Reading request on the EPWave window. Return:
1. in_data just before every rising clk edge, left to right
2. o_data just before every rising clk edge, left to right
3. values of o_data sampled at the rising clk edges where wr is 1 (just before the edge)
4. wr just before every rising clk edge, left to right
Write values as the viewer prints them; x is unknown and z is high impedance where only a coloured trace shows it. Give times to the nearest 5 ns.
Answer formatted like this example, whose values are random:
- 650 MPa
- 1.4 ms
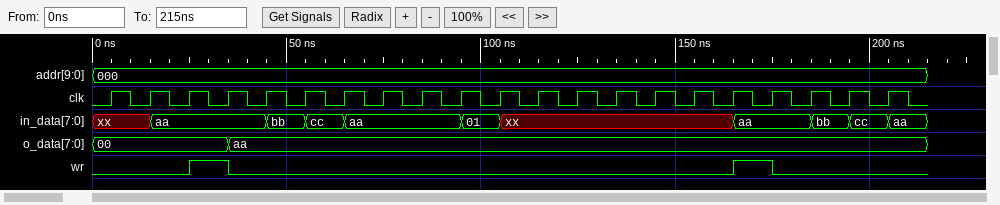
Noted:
- xx, xx, aa, aa, aa, bb, cc, aa, aa, aa, 01, xx, xx, xx, xx, xx, xx, aa, aa, bb, cc
- 00, 00, 00, 00, aa, aa, aa, aa, aa, aa, aa, aa, aa, aa, aa, aa, aa, aa, aa, aa, aa
- 00, aa
- 0 0 0 1 0 0 0 0 0 0 0 0 0 0 0 0 0 1 0 0 0
